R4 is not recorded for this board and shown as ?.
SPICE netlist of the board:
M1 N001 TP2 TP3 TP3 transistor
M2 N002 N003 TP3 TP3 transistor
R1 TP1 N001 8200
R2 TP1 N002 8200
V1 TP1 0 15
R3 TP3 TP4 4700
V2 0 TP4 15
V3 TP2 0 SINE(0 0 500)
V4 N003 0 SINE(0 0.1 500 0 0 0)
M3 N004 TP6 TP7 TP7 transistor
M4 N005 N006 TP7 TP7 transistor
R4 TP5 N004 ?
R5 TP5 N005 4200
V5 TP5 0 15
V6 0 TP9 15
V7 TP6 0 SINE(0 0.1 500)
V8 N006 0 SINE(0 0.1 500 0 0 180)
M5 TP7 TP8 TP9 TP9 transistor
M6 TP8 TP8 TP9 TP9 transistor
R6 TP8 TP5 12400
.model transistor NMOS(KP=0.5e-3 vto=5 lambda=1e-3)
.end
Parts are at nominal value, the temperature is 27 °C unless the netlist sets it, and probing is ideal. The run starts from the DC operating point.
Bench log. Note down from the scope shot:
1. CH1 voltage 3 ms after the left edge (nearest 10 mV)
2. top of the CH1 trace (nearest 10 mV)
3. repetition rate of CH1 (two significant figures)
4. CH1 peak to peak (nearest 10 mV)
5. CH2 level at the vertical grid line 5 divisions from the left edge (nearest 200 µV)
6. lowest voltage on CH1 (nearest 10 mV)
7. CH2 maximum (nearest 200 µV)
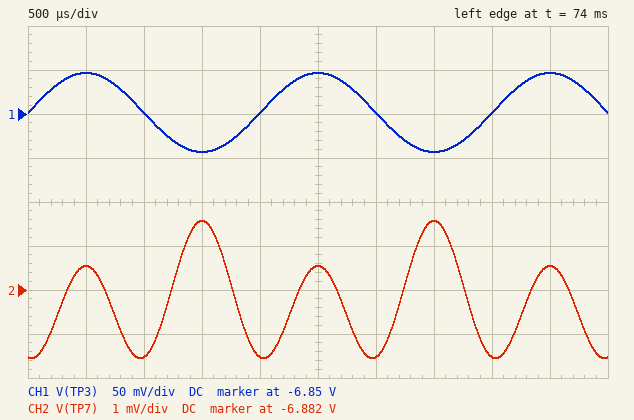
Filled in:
-6.85 V
-6.80 V
500 Hz
90 mV
-6.8814 V
-6.89 V
-6.8804 V
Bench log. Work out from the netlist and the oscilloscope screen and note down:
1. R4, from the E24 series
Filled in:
10 kΩ
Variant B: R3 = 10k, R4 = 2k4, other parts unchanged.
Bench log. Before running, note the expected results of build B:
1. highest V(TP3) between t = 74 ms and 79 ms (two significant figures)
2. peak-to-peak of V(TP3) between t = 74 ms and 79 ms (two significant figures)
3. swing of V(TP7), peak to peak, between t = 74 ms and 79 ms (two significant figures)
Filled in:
-6.3 V
93 mV
2.8 mV
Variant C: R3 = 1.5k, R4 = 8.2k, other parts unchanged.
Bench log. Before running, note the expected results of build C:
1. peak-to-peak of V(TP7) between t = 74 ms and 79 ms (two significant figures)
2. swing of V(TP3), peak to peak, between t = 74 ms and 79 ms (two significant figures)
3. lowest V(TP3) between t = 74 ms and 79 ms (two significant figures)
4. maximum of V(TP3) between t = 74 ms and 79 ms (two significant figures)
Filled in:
3.0 mV
82 mV
-8.1 V
-8.0 V
